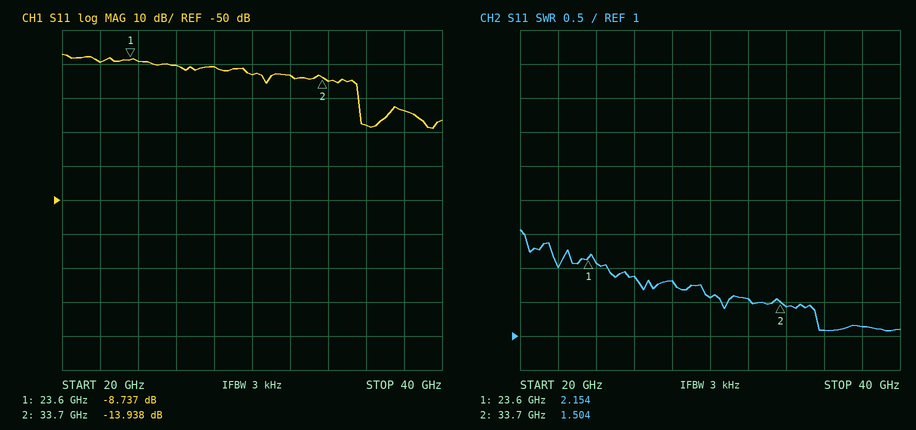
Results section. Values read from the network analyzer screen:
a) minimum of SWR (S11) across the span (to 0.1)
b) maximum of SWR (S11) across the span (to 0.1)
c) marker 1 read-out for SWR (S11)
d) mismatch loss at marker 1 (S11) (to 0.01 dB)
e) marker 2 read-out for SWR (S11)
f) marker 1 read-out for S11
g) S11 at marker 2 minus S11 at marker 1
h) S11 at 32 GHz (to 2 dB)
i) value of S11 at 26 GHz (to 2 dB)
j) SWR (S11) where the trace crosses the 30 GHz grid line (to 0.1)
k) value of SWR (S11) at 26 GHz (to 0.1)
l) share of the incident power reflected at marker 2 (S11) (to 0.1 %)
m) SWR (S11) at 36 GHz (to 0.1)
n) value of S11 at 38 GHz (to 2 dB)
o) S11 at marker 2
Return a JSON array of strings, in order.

["1.1", "2.6", "2.154", "0.62 dB", "1.504", "-8.737 dB", "-5.201 dB", "-14 dB", "-10 dB", "1.6", "1.9", "4.0 %", "1.1", "-24 dB", "-13.938 dB"]
